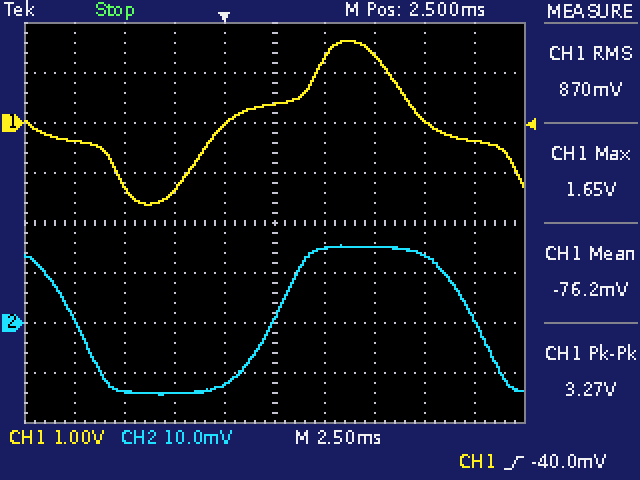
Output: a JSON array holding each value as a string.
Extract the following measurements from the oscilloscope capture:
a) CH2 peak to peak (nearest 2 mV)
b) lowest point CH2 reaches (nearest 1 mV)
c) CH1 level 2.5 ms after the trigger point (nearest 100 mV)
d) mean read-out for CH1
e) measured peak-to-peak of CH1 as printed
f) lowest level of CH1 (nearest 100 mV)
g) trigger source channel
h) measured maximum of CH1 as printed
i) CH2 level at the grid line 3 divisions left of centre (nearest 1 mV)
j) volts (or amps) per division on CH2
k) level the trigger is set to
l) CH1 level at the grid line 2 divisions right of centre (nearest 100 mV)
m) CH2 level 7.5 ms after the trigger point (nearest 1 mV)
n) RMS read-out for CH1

["30 mV", "-14 mV", "400 mV", "-76.2 mV", "3.27 V", "-1.6 V", "CH1", "1.65 V", "-14 mV", "10 mV", "-40.0 mV", "1.4 V", "15 mV", "870 mV"]
